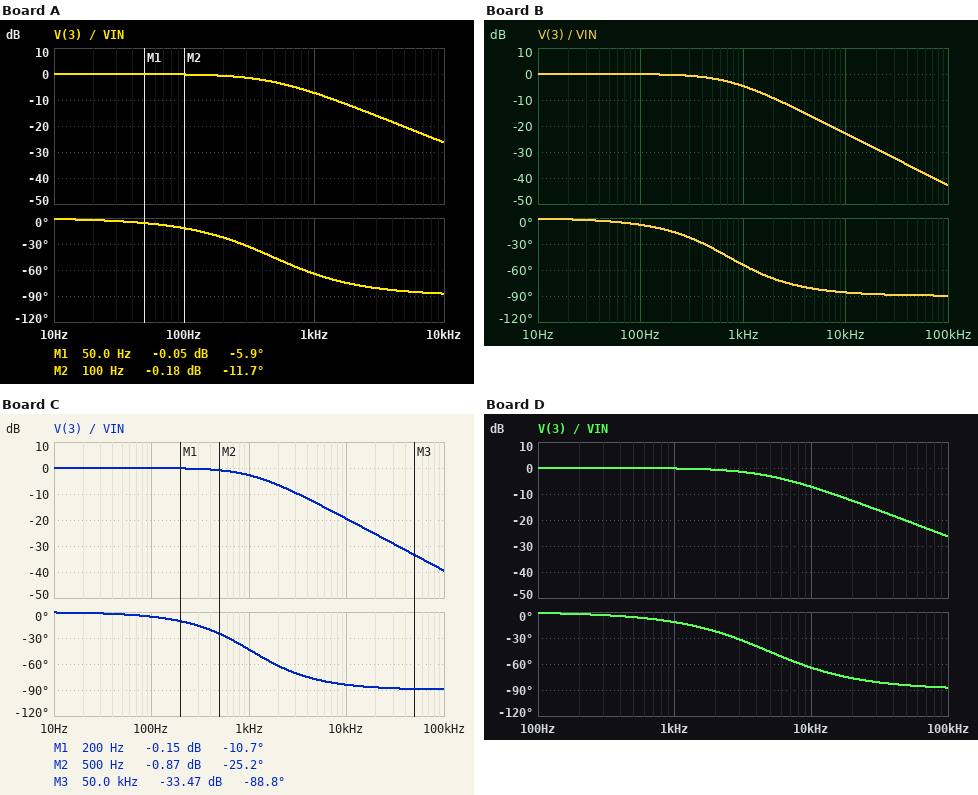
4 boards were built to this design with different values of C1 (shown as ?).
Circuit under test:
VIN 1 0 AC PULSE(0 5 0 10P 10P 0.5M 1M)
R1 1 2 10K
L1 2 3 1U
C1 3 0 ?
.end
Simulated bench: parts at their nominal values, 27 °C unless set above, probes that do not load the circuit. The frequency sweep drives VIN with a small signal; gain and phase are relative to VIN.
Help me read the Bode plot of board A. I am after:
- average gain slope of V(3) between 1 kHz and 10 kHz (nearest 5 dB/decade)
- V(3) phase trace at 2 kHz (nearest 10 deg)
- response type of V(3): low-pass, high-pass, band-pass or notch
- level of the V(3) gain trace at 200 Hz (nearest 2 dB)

-20 dB/decade
-80 deg
low-pass
0 dB
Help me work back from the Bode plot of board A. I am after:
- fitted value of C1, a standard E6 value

33 nF
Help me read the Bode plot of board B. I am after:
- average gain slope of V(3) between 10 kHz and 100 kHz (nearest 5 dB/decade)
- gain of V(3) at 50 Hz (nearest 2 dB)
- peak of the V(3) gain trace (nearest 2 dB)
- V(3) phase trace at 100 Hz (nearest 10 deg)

-20 dB/decade
0 dB
0 dB
-10 deg
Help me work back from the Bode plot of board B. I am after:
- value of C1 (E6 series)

22 nF
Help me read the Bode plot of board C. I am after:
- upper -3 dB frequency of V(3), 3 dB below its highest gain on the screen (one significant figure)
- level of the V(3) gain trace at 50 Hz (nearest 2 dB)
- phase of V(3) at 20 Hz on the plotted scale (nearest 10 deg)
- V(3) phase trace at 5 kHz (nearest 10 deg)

1 kHz
0 dB
0 deg
-80 deg
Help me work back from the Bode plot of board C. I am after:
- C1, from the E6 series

15 nF
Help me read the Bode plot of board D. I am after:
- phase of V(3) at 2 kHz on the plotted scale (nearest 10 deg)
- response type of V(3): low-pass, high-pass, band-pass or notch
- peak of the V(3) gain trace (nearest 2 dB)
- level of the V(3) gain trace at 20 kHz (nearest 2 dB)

-20 deg
low-pass
0 dB
-12 dB
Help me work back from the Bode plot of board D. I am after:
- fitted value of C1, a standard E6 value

3.3 nF
